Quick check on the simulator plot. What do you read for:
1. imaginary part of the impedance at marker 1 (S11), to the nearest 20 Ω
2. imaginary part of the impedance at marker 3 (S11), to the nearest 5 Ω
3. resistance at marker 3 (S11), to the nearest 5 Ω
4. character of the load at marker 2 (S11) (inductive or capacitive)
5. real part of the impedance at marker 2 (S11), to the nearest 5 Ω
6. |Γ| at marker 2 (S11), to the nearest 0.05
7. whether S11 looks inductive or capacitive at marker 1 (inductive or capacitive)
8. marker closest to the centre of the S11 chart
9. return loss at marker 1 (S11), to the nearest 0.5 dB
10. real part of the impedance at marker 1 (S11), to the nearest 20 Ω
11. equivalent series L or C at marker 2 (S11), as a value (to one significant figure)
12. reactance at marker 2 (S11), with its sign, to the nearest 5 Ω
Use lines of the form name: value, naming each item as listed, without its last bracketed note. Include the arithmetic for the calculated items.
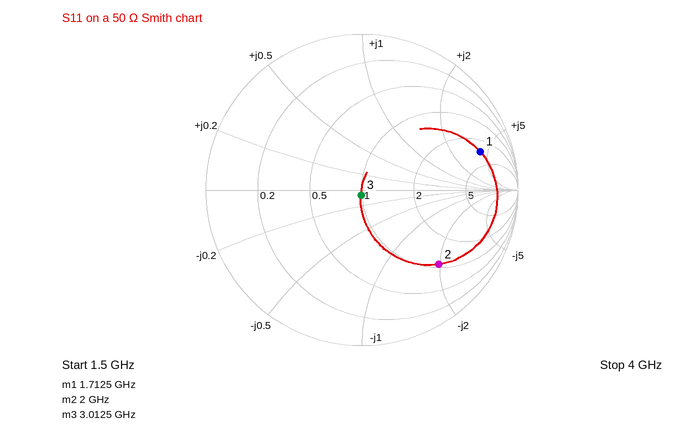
imaginary part of the impedance at marker 1 (S11), to the nearest 20 Ω: +200 Ω
imaginary part of the impedance at marker 3 (S11), to the nearest 5 Ω: -5 Ω
resistance at marker 3 (S11), to the nearest 5 Ω: 50 Ω
character of the load at marker 2 (S11): capacitive
real part of the impedance at marker 2 (S11), to the nearest 5 Ω: 55 Ω
|Γ| at marker 2 (S11), to the nearest 0.05: 0.70
whether S11 looks inductive or capacitive at marker 1: inductive
marker closest to the centre of the S11 chart: marker 3
return loss at marker 1 (S11), to the nearest 0.5 dB: 2.0 dB
real part of the impedance at marker 1 (S11), to the nearest 20 Ω: 160 Ω
equivalent series L or C at marker 2 (S11), as a value: C = 1/(2π × 2 GHz × 100 Ω) ≈ 796 fF, so 800 fF to one significant figure
reactance at marker 2 (S11), with its sign, to the nearest 5 Ω: -100 Ω
